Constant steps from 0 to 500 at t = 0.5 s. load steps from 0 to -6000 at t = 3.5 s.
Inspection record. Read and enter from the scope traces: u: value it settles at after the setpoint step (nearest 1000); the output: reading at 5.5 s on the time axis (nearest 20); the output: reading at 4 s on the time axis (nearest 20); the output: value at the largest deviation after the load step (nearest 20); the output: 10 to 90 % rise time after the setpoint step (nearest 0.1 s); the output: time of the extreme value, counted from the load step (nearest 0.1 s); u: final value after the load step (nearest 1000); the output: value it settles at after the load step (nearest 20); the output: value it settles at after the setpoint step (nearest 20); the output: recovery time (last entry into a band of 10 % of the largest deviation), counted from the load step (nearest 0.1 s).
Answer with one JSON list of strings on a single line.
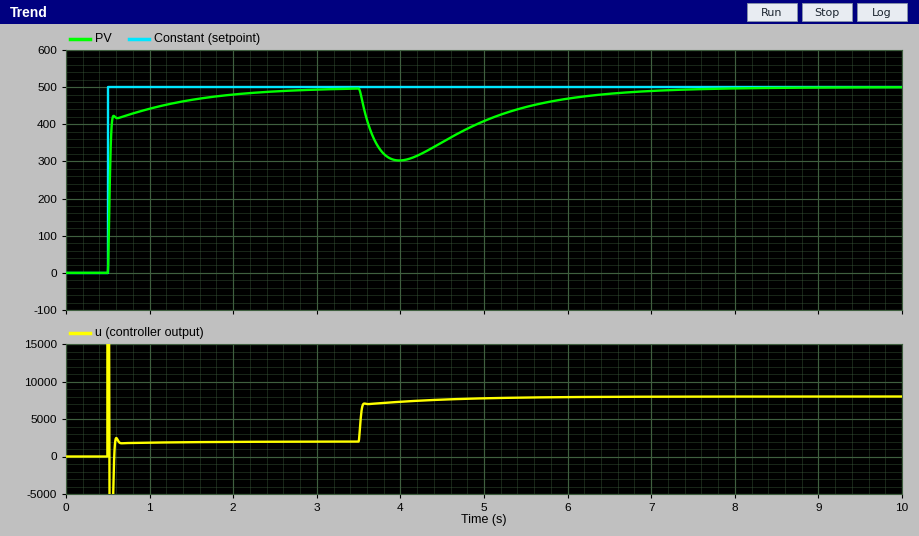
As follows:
["2000", "440", "300", "300", "0.6 s", "0.5 s", "8000", "500", "500", "2.9 s"]
